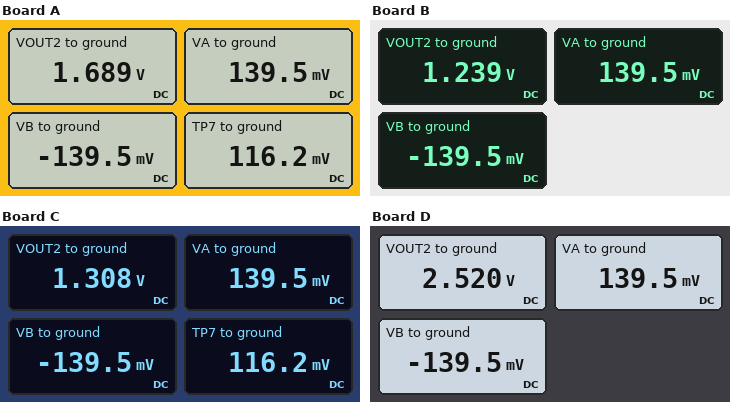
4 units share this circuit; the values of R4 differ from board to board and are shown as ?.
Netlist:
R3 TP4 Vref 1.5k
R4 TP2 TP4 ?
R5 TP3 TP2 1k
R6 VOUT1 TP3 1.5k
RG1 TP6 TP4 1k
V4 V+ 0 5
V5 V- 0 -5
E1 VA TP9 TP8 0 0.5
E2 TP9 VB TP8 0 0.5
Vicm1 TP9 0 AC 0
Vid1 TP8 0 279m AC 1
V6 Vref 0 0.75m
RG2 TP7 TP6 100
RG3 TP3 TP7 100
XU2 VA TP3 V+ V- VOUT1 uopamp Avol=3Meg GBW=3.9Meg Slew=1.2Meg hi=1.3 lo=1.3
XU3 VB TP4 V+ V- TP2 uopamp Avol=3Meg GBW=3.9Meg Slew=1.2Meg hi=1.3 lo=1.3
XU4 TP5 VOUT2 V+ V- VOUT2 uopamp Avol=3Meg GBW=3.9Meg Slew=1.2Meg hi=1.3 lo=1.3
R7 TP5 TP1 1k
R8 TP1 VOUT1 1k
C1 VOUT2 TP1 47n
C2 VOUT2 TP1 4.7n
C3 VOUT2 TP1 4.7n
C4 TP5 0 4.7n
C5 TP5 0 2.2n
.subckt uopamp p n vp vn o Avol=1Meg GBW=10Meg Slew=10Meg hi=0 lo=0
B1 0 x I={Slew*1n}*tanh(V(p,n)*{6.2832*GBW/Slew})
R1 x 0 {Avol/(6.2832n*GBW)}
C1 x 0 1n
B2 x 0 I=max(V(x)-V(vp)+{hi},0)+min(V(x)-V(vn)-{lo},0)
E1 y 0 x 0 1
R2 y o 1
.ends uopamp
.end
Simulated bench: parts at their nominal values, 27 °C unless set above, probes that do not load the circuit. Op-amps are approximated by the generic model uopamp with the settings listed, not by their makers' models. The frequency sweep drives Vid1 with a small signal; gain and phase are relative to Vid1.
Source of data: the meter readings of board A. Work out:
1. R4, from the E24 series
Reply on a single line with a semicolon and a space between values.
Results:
1.6 kΩ
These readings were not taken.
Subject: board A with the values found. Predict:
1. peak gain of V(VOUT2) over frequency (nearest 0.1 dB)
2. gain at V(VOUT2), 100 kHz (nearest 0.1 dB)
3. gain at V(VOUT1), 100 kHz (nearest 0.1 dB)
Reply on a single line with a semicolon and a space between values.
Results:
19.3 dB; -28.3 dB; 15.5 dB
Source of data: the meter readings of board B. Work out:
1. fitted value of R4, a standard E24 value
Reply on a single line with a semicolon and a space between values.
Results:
680 Ω
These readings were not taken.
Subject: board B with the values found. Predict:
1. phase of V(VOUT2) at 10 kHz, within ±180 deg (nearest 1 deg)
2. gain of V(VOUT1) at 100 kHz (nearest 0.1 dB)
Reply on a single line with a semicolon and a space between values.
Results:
-123 deg; 12.9 dB
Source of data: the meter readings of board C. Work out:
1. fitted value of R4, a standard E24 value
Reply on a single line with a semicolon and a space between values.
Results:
820 Ω
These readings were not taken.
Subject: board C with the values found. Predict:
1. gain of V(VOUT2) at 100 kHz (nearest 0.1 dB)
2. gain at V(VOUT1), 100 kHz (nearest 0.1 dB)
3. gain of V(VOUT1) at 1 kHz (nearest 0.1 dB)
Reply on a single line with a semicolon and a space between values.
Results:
-30.4 dB; 13.3 dB; 13.4 dB
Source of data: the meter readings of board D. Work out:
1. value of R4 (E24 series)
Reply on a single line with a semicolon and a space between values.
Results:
3.3 kΩ
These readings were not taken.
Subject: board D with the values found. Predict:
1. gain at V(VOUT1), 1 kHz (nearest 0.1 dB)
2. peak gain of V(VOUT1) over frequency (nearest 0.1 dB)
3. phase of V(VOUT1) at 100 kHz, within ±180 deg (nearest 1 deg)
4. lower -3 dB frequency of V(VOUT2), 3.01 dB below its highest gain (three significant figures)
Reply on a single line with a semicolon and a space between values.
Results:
19.1 dB; 19.1 dB; -18 deg; 2.58 kHz
